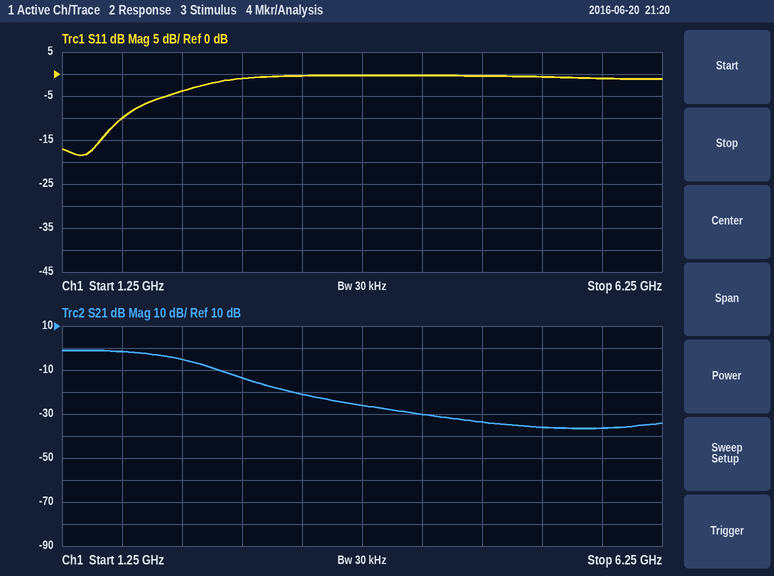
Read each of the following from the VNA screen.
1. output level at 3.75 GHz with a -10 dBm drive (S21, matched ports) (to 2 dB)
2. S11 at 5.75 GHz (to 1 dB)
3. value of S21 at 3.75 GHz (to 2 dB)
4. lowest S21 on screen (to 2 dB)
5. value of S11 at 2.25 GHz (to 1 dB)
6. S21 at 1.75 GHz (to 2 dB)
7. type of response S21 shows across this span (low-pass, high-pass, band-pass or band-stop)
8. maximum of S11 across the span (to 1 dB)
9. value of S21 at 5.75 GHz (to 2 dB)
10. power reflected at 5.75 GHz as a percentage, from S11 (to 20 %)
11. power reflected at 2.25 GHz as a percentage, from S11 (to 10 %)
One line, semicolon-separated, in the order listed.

-36 dBm; -1 dB; -26 dB; -36 dB; -4 dB; -2 dB; low-pass; 0 dB; -36 dB; 80 %; 40 %
